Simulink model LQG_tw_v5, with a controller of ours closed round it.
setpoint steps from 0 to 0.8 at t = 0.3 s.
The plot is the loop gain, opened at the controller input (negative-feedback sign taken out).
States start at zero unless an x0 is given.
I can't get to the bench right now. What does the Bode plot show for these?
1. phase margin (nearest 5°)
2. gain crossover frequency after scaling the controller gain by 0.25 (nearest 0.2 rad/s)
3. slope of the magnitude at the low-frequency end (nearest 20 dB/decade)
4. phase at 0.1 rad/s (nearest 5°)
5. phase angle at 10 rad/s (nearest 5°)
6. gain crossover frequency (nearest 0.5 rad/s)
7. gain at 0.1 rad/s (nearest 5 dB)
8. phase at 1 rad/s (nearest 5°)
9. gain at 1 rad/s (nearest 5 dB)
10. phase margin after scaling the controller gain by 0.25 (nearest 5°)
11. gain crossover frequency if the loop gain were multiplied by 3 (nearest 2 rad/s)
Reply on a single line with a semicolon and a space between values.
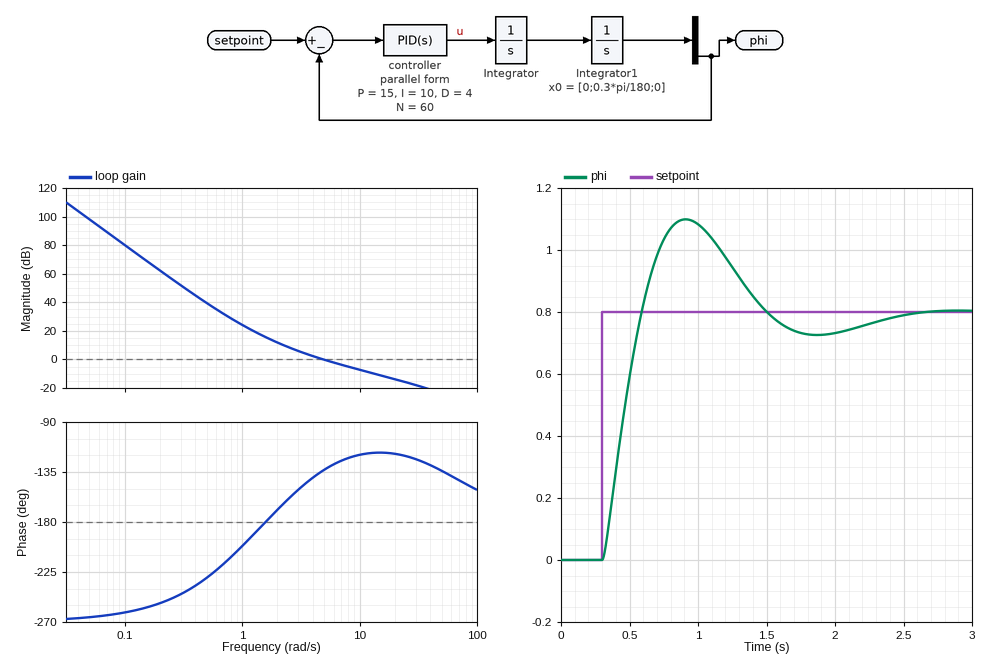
45°; 2.0 rad/s; -60 dB/decade; -260°; -120°; 5.0 rad/s; 80 dB; -200°; 25 dB; 10°; 12 rad/s
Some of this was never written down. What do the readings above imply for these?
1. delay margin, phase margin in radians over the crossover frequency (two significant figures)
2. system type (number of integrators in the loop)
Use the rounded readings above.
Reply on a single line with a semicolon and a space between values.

0.16 s; 3
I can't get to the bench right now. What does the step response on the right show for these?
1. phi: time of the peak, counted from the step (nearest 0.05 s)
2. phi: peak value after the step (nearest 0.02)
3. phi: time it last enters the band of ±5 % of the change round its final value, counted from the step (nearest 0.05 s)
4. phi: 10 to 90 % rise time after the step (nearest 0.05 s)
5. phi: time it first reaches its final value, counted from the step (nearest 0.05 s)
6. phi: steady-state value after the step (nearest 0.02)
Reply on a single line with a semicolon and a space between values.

0.60 s; 1.10; 1.95 s; 0.20 s; 0.30 s; 0.80
